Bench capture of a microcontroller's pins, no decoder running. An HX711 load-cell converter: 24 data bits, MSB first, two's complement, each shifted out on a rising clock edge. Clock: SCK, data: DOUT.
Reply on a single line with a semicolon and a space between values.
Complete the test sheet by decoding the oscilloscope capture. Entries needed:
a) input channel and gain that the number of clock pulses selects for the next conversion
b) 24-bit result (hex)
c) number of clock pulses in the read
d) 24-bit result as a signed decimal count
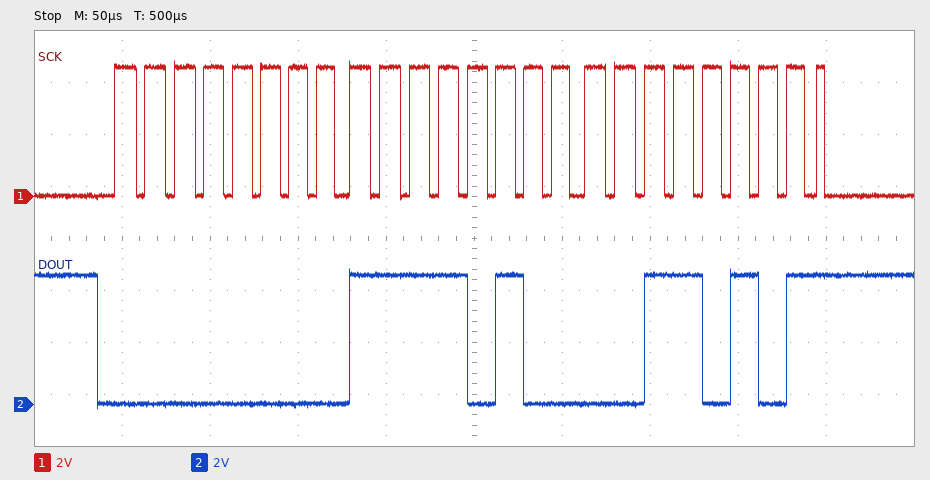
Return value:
channel A, gain 128; 0x00F435; 25; 62517
